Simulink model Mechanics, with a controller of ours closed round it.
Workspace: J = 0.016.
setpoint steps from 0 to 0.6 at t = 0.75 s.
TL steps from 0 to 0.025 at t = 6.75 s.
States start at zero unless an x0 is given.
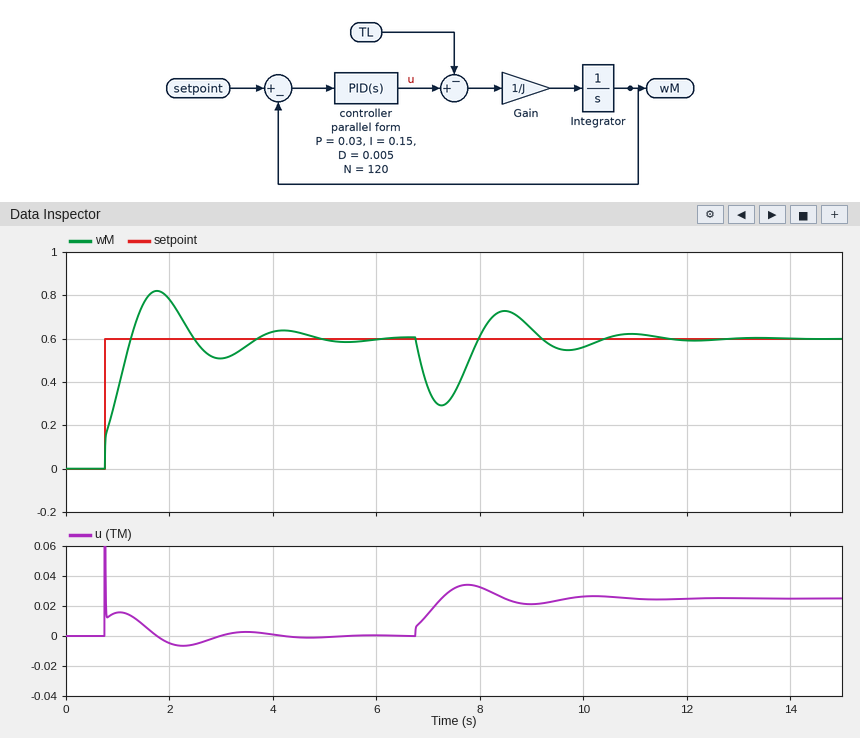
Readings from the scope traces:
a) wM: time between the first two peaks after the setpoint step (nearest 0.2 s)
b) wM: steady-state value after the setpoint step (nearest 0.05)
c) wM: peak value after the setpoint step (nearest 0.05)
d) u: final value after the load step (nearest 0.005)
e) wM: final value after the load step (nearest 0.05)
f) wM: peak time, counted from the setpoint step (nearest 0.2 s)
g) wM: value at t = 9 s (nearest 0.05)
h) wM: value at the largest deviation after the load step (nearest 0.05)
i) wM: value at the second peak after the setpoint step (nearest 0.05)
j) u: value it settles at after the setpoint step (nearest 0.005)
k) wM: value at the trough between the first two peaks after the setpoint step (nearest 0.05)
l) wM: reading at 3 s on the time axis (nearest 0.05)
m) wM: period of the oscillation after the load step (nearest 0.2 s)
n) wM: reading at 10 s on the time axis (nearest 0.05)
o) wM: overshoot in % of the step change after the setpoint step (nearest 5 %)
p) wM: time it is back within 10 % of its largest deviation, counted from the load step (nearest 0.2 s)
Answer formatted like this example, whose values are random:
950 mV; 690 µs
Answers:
2.4 s; 0.60; 0.80; 0.025; 0.60; 1.0 s; 0.65; 0.30; 0.65; 0.000; 0.50; 0.50; 2.4 s; 0.55; 35 %; 3.4 s
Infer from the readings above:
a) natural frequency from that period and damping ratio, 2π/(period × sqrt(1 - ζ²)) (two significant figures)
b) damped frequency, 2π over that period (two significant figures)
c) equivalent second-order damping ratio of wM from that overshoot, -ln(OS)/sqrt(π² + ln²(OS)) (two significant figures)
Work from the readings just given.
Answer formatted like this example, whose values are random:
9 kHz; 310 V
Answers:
2.8 rad/s; 2.6 rad/s; 0.32
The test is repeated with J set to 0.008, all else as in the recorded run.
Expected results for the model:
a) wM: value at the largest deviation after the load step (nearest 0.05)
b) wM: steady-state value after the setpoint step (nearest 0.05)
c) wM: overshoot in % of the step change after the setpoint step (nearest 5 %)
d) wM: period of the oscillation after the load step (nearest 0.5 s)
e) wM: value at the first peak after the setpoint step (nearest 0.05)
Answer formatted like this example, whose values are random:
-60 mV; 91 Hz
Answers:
0.25; 0.60; 25 %; 2.0 s; 0.75
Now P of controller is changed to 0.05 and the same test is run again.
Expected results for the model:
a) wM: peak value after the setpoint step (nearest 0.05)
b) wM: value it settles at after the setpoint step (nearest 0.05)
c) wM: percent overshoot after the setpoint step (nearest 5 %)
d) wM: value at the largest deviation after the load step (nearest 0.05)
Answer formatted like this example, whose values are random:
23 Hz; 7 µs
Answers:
0.75; 0.60; 25 %; 0.35
